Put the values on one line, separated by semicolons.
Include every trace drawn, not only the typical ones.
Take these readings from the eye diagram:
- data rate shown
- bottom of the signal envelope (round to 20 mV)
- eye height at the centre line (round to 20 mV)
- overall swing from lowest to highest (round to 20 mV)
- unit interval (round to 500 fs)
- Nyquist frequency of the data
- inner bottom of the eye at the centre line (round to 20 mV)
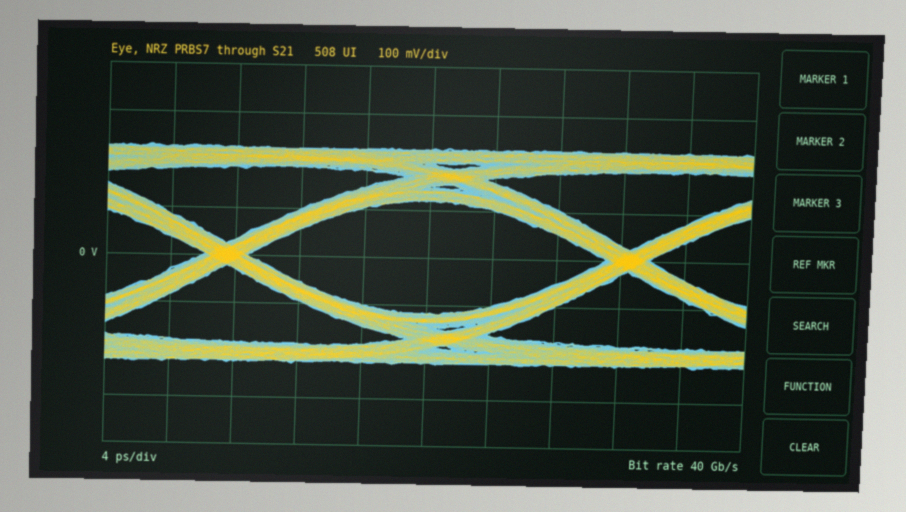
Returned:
40 Gb/s; -220 mV; 240 mV; 460 mV; 25.0 ps; 20 GHz; -120 mV
